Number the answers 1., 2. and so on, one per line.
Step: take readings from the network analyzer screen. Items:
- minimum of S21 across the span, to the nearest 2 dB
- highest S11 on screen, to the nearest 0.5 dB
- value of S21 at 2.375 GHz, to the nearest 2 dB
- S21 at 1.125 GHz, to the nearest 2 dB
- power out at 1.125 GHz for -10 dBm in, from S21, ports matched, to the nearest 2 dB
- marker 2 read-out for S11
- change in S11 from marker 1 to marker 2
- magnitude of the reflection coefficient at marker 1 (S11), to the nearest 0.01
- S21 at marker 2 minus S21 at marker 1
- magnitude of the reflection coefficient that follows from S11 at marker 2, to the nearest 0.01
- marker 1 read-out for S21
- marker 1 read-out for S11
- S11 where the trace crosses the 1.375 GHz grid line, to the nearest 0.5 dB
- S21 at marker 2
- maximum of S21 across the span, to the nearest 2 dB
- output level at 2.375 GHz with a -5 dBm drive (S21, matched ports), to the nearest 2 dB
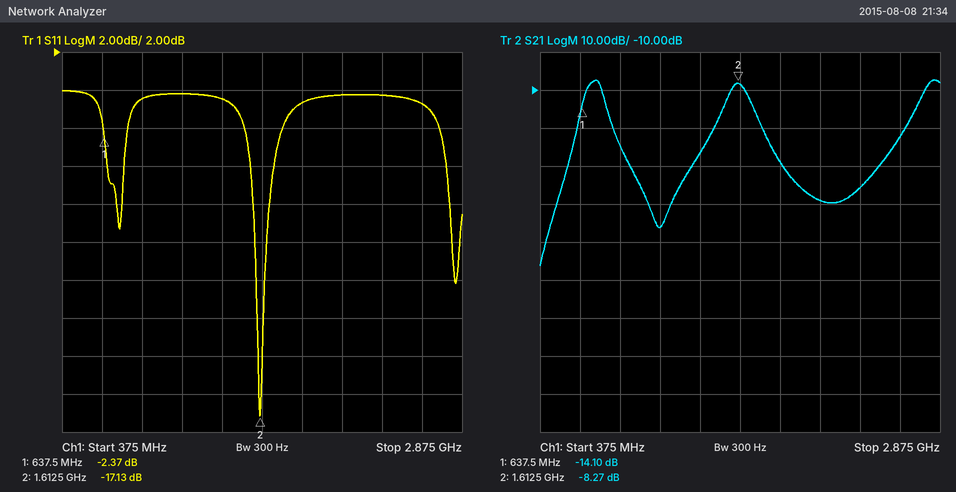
1. -56 dB
2. 0.0 dB
3. -36 dB
4. -46 dB
5. -56 dBm
6. -17.13 dB
7. -14.76 dB
8. 0.76
9. 5.83 dB
10. 0.14
11. -14.10 dB
12. -2.37 dB
13. -0.5 dB
14. -8.27 dB
15. -8 dB
16. -40 dBm
